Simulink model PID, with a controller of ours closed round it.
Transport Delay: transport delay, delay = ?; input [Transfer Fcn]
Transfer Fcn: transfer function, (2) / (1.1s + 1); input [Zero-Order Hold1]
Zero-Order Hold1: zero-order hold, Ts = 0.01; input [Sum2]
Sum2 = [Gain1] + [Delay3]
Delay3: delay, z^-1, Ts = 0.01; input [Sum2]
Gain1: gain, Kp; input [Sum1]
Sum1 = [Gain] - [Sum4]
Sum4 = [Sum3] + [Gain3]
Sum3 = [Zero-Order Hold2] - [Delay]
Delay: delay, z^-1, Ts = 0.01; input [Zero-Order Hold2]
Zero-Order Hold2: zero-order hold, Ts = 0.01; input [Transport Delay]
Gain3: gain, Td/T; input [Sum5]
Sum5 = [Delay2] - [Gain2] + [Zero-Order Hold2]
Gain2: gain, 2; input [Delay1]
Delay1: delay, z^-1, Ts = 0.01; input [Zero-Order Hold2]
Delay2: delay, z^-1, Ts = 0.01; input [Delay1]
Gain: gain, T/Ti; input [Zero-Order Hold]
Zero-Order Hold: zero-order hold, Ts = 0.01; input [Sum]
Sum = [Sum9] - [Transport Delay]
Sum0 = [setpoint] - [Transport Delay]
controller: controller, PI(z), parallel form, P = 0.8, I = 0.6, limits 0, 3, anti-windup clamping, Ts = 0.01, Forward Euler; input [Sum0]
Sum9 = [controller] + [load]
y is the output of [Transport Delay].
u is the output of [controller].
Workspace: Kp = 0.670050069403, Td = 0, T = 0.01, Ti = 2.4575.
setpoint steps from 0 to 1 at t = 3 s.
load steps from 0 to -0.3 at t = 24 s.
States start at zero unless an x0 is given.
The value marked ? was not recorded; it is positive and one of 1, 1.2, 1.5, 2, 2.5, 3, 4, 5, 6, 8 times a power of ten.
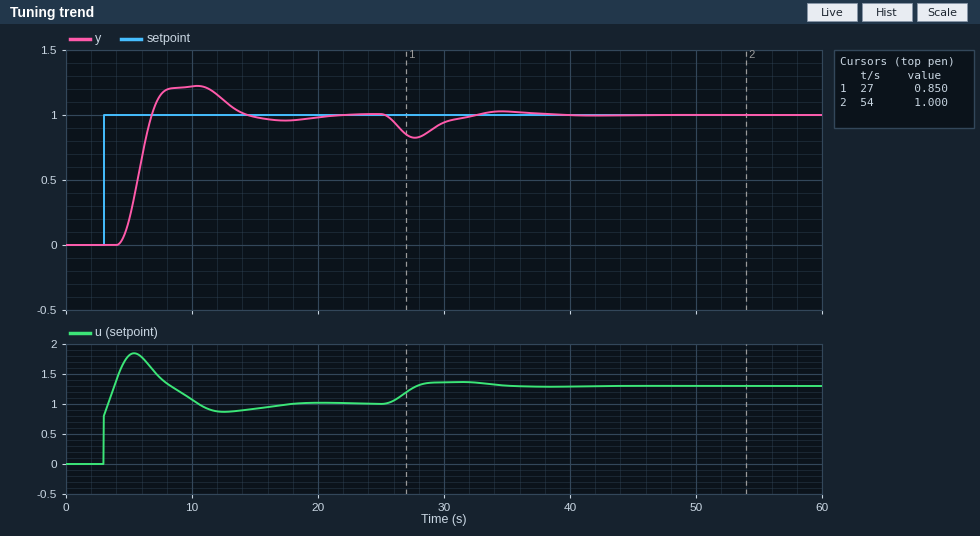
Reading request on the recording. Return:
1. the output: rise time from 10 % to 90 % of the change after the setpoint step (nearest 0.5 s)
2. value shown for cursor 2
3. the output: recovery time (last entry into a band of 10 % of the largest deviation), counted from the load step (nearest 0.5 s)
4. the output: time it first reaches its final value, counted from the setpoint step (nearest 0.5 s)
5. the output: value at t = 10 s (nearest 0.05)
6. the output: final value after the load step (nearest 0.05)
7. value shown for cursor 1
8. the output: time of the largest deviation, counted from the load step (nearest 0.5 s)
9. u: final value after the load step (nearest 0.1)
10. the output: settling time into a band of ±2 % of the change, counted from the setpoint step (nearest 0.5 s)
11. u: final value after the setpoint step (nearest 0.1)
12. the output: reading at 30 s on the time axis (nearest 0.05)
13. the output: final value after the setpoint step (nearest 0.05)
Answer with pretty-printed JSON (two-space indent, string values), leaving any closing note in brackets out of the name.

{
  "the output: rise time from 10 % to 90 % of the change after the setpoint step": "2.0 s",
  "value shown for cursor 2": "1.000",
  "the output: recovery time (last entry into a band of 10 % of the largest deviation), counted from the load step": "12.5 s",
  "the output: time it first reaches its final value, counted from the setpoint step": "4.0 s",
  "the output: value at t = 10 s": "1.20",
  "the output: final value after the load step": "1.00",
  "value shown for cursor 1": "0.850",
  "the output: time of the largest deviation, counted from the load step": "3.5 s",
  "u: final value after the load step": "1.3",
  "the output: settling time into a band of ±2 % of the change, counted from the setpoint step": "17.0 s",
  "u: final value after the setpoint step": "1.0",
  "the output: reading at 30 s on the time axis": "0.95",
  "the output: final value after the setpoint step": "1.00"
}
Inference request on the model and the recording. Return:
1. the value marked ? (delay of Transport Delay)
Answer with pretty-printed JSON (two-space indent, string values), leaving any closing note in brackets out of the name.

{
  "the value marked ?": "1"
}
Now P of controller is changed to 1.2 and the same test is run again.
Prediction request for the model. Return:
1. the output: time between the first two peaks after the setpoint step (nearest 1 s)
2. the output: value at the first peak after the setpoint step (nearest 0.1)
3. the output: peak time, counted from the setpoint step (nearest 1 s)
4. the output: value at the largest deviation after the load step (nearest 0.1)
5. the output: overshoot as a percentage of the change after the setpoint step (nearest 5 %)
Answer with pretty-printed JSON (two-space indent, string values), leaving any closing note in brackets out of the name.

{
  "the output: time between the first two peaks after the setpoint step": "4 s",
  "the output: value at the first peak after the setpoint step": "1.3",
  "the output: peak time, counted from the setpoint step": "4 s",
  "the output: value at the largest deviation after the load step": "0.8",
  "the output: overshoot as a percentage of the change after the setpoint step": "25 %"
}
